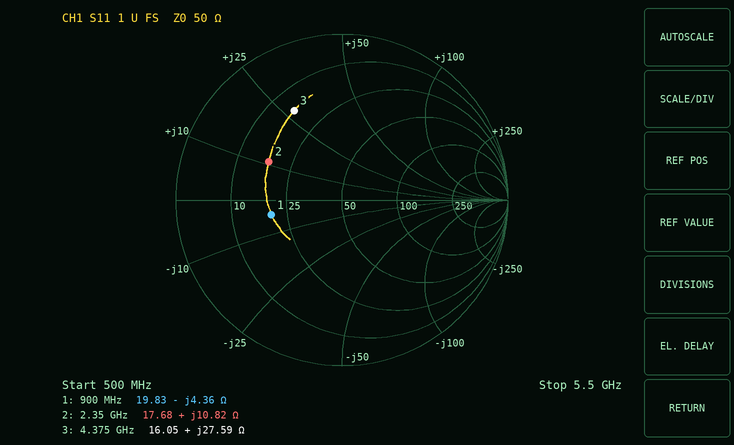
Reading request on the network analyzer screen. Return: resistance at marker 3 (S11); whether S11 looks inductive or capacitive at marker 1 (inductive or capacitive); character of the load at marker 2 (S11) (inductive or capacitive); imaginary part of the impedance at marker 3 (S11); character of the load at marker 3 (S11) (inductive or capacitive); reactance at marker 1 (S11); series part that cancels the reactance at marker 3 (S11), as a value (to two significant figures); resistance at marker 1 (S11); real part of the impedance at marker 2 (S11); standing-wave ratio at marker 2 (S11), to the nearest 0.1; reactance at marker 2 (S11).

16.05 Ω
capacitive
inductive
+27.59 Ω
inductive
-4.36 Ω
1.3 pF
19.83 Ω
17.68 Ω
3.0
+10.82 Ω
